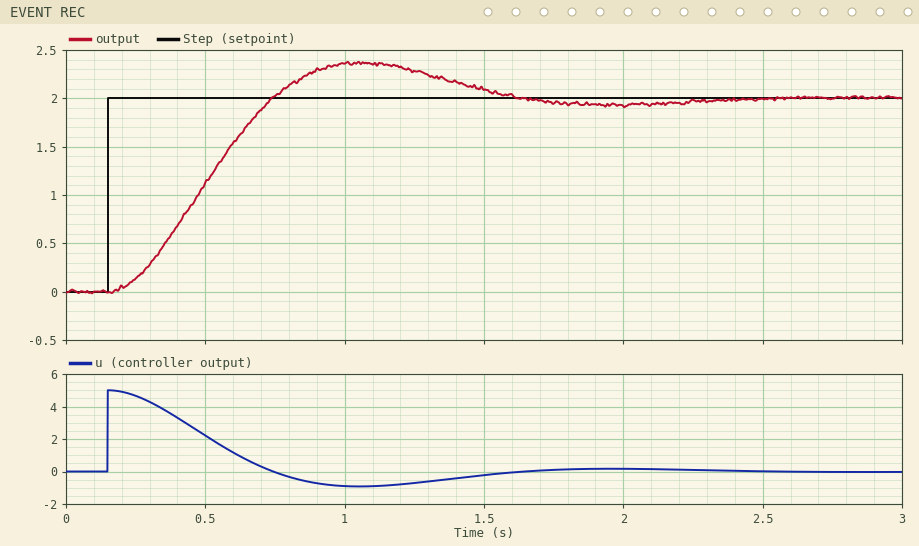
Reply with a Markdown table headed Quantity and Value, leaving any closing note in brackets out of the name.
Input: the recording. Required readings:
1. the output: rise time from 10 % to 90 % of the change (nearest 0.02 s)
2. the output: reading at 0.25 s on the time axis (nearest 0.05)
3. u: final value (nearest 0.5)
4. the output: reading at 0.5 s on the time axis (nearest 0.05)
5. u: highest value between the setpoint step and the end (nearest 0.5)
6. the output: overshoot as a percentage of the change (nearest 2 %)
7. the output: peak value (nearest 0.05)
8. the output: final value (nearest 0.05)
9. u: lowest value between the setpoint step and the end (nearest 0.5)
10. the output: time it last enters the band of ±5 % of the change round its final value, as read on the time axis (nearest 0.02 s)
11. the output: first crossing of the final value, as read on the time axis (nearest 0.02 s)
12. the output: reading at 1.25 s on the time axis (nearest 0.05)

| Quantity | Value |
|---|---|
| the output: rise time from 10 % to 90 % of the change | 0.40 s |
| the output: reading at 0.25 s on the time axis | 0.15 |
| u: final value | 0.0 |
| the output: reading at 0.5 s on the time axis | 1.10 |
| u: highest value between the setpoint step and the end | 5.0 |
| the output: overshoot as a percentage of the change | 18 % |
| the output: peak value | 2.35 |
| the output: final value | 2.00 |
| u: lowest value between the setpoint step and the end | -1.0 |
| the output: time it last enters the band of ±5 % of the change round its final value, as read on the time axis | 1.48 s |
| the output: first crossing of the final value, as read on the time axis | 0.74 s |
| the output: reading at 1.25 s on the time axis | 2.30 |
